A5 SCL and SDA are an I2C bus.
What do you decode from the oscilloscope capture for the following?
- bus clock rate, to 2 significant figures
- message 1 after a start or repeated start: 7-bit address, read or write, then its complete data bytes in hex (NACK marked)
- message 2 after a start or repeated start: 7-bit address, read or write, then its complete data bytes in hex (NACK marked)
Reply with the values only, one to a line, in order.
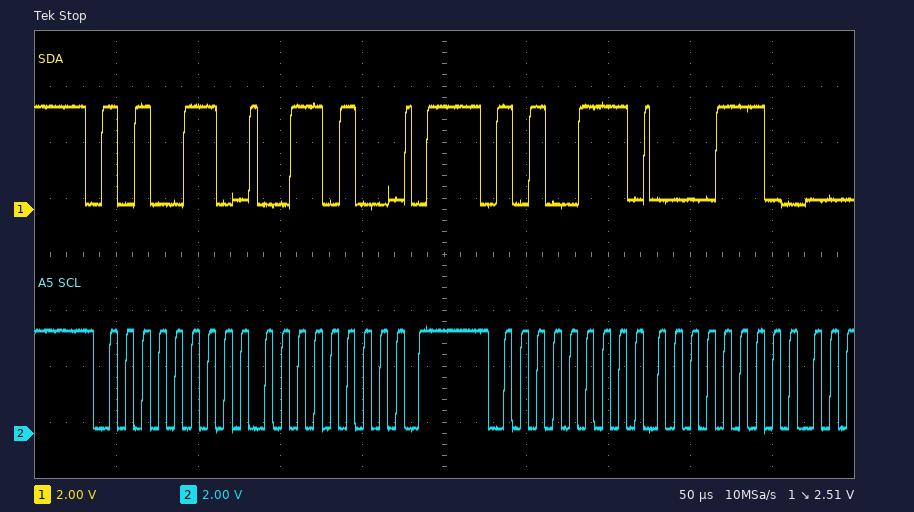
100 kHz
0x53 write: 34
0x53 read: 0E
